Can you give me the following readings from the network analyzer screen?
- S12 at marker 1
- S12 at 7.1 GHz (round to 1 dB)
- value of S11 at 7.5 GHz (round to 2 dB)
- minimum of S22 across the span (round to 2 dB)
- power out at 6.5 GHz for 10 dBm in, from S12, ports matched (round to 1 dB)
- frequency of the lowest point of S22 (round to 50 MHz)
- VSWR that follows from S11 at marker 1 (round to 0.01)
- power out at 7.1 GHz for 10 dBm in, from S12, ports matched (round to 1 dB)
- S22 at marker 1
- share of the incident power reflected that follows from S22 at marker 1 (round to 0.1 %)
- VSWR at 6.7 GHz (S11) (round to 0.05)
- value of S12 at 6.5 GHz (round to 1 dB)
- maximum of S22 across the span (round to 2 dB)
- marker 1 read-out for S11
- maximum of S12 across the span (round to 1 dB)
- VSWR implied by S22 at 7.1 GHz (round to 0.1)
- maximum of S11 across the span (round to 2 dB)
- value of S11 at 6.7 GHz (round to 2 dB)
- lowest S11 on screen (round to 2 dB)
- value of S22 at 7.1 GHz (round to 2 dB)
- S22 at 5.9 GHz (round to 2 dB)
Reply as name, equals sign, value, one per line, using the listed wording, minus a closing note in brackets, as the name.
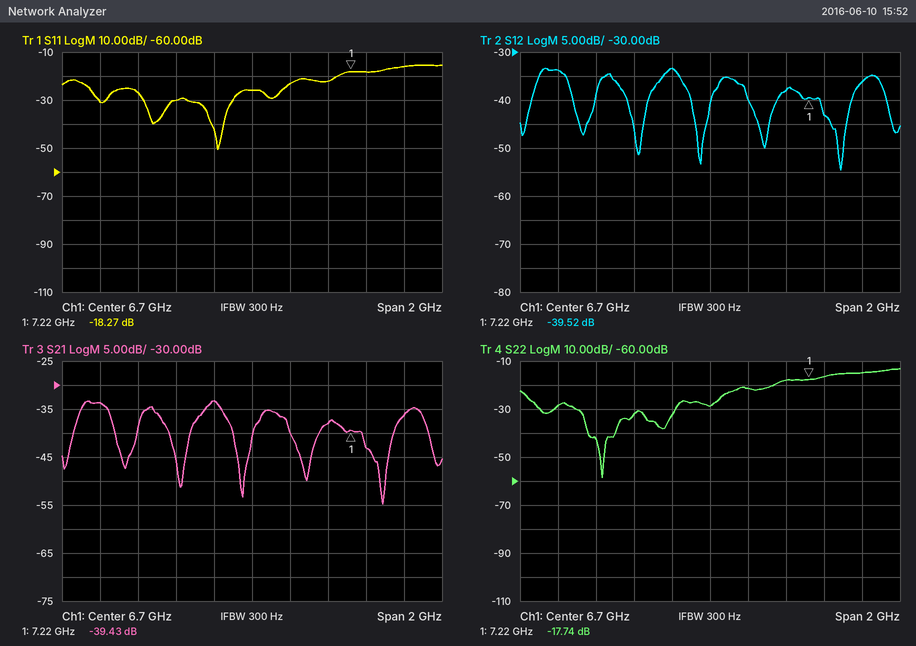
S12 at marker 1 = -39.52 dB
S12 at 7.1 GHz = -38 dB
value of S11 at 7.5 GHz = -16 dB
minimum of S22 across the span = -58 dB
power out at 6.5 GHz for 10 dBm in, from S12, ports matched = -23 dBm
frequency of the lowest point of S22 = 6.15 GHz
VSWR that follows from S11 at marker 1 = 1.28
power out at 7.1 GHz for 10 dBm in, from S12, ports matched = -28 dBm
S22 at marker 1 = -17.74 dB
share of the incident power reflected that follows from S22 at marker 1 = 1.7 %
VSWR at 6.7 GHz (S11) = 1.10
value of S12 at 6.5 GHz = -33 dB
maximum of S22 across the span = -14 dB
marker 1 read-out for S11 = -18.27 dB
maximum of S12 across the span = -33 dB
VSWR implied by S22 at 7.1 GHz = 1.3
maximum of S11 across the span = -16 dB
value of S11 at 6.7 GHz = -26 dB
lowest S11 on screen = -50 dB
value of S22 at 7.1 GHz = -18 dB
S22 at 5.9 GHz = -28 dB
